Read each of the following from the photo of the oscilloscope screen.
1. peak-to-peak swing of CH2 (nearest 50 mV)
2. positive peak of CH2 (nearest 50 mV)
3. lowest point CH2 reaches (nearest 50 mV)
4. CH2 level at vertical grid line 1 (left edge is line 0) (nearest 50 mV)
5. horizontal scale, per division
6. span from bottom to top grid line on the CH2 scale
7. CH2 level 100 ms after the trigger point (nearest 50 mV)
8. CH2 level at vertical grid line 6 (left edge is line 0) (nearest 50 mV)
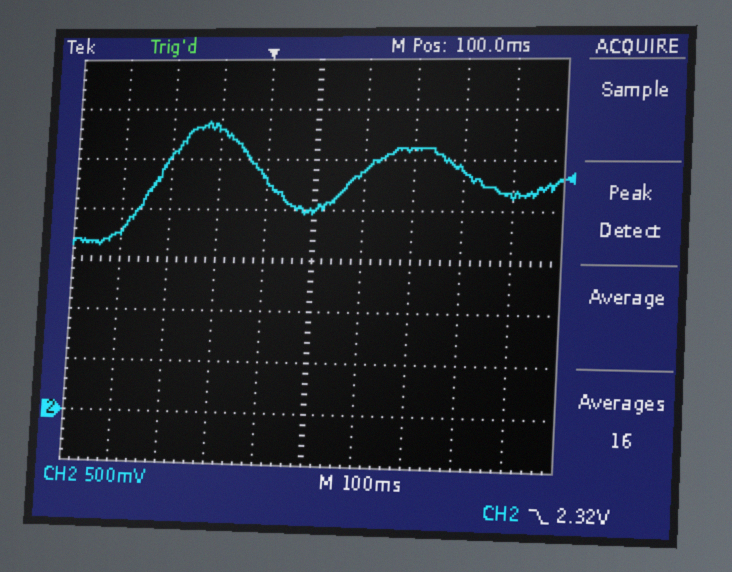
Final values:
1.25 V
2.90 V
1.65 V
1.80 V
100 ms
4 V
2.00 V
2.40 V
